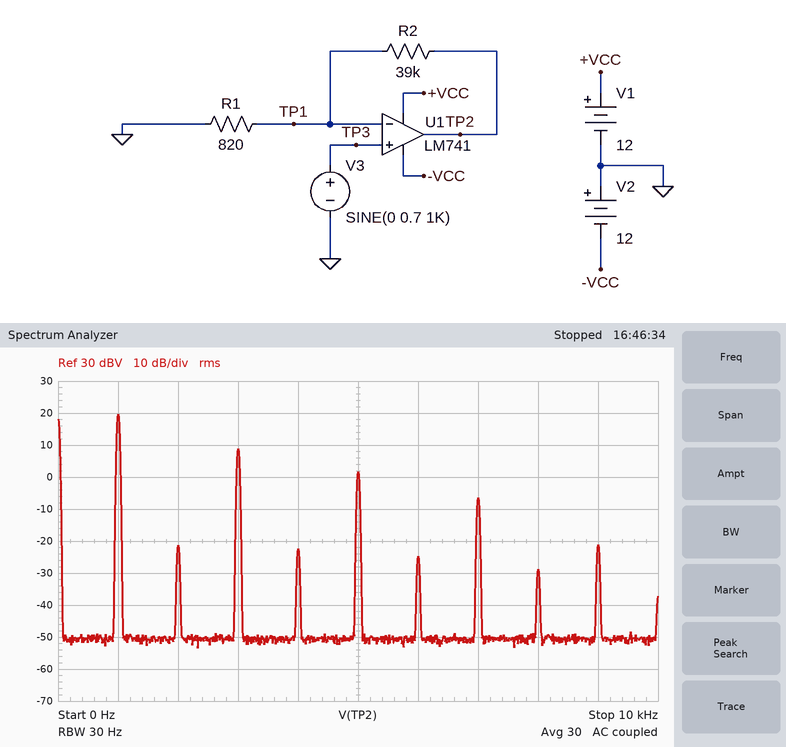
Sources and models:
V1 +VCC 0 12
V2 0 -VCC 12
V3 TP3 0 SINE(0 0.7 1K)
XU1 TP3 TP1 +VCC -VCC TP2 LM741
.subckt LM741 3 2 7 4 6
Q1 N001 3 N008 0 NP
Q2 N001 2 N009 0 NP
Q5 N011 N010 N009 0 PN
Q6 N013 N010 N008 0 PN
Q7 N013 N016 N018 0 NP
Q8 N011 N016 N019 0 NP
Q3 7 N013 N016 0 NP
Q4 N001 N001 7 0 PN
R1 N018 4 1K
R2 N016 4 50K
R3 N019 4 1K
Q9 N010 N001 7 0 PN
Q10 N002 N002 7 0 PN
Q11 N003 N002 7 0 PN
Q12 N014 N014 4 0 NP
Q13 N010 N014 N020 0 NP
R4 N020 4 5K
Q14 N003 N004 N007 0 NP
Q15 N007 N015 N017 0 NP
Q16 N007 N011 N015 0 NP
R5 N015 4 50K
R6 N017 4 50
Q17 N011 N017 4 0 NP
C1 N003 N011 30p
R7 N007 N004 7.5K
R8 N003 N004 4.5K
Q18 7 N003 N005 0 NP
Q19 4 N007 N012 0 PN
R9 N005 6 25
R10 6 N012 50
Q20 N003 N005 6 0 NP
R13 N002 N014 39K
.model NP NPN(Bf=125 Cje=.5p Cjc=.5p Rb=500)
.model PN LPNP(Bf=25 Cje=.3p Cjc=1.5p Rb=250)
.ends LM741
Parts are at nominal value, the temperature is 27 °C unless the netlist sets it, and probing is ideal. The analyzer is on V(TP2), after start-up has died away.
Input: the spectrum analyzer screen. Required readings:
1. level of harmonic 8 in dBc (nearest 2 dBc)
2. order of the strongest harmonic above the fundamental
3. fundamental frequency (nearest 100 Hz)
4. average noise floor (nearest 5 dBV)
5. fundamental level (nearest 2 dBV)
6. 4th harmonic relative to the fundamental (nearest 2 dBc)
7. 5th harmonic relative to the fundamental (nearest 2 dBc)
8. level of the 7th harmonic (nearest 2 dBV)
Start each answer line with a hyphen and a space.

- -48 dBc
- 3
- 1.0 kHz
- -50 dBV
- 20 dBV
- -42 dBc
- -18 dBc
- -6 dBV
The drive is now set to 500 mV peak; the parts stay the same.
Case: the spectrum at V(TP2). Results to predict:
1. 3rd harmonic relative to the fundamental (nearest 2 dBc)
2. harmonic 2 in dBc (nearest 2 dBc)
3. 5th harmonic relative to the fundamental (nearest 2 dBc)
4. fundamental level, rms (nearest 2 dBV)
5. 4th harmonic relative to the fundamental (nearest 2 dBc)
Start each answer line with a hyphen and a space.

- -12 dBc
- -38 dBc
- -24 dBc
- 20 dBV
- -40 dBc
